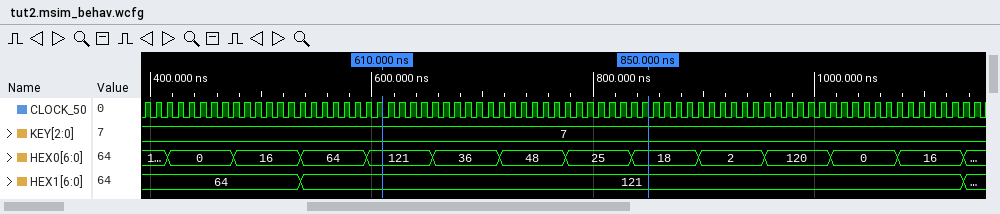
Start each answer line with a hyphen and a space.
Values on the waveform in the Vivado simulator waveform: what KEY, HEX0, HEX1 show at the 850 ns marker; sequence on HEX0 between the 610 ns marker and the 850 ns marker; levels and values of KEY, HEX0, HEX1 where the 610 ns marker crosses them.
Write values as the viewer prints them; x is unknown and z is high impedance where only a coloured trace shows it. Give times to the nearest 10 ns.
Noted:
- KEY=7, HEX0=18, HEX1=121
- 121, 36, 48, 25, 18
- KEY=7, HEX0=121, HEX1=121
